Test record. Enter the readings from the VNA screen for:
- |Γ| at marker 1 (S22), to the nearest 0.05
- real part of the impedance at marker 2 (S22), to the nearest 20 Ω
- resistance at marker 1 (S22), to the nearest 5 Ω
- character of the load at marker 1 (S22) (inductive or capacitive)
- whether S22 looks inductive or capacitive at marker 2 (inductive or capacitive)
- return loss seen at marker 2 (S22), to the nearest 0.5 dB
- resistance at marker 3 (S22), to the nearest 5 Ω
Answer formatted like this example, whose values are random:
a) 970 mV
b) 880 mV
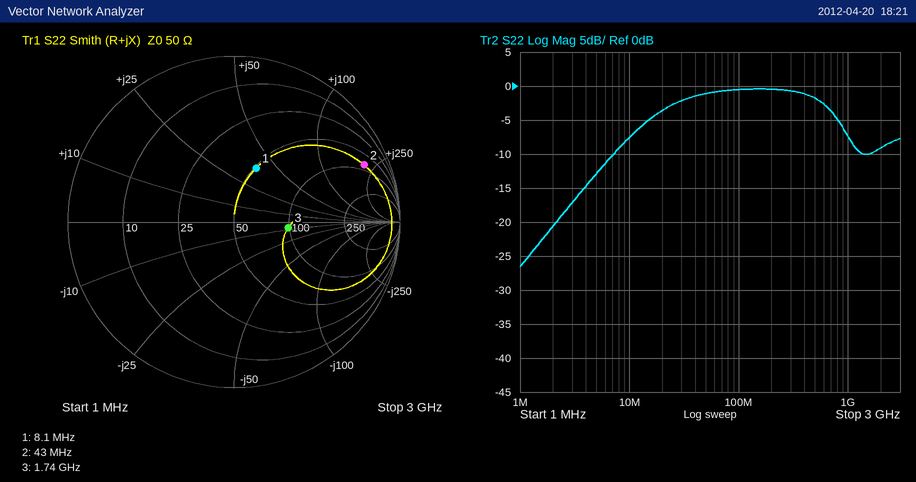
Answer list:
a) 0.35
b) 80 Ω
c) 50 Ω
d) inductive
e) inductive
f) 1.5 dB
g) 100 Ω
